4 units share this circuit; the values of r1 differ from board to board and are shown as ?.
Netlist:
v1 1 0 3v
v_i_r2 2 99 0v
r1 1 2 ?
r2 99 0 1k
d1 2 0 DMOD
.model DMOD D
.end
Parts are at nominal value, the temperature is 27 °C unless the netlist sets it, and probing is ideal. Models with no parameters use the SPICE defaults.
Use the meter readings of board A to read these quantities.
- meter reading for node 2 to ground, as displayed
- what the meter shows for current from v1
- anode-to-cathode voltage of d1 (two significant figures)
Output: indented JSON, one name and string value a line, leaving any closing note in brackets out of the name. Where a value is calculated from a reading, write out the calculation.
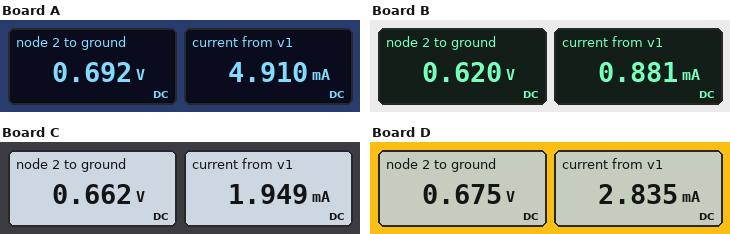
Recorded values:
{
  "meter reading for node 2 to ground, as displayed": "0.692 V",
  "what the meter shows for current from v1": "4.910 mA",
  "anode-to-cathode voltage of d1": "692 mV = 690 mV"
}
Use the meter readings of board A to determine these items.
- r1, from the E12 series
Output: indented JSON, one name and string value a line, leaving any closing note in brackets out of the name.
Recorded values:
{
  "r1, from the E12 series": "470 Ω"
}
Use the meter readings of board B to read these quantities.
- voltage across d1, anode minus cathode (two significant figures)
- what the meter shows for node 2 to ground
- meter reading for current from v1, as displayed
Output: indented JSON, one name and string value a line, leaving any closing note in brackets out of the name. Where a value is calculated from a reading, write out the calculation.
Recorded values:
{
  "voltage across d1, anode minus cathode": "620 mV = 620 mV",
  "what the meter shows for node 2 to ground": "0.620 V",
  "meter reading for current from v1, as displayed": "0.881 mA"
}
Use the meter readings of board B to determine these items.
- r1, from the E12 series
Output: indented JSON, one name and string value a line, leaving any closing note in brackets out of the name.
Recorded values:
{
  "r1, from the E12 series": "2.7 kΩ"
}
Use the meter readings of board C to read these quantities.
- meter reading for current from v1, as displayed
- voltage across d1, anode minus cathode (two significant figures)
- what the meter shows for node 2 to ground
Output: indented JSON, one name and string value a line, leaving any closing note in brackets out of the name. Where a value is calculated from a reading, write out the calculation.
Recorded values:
{
  "meter reading for current from v1, as displayed": "1.949 mA",
  "voltage across d1, anode minus cathode": "662 mV = 660 mV",
  "what the meter shows for node 2 to ground": "0.662 V"
}
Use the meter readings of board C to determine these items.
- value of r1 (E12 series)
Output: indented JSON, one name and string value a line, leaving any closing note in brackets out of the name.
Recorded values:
{
  "value of r1": "1.2 kΩ"
}
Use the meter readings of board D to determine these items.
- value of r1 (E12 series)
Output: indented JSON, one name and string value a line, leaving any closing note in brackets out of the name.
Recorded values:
{
  "value of r1": "820 Ω"
}
